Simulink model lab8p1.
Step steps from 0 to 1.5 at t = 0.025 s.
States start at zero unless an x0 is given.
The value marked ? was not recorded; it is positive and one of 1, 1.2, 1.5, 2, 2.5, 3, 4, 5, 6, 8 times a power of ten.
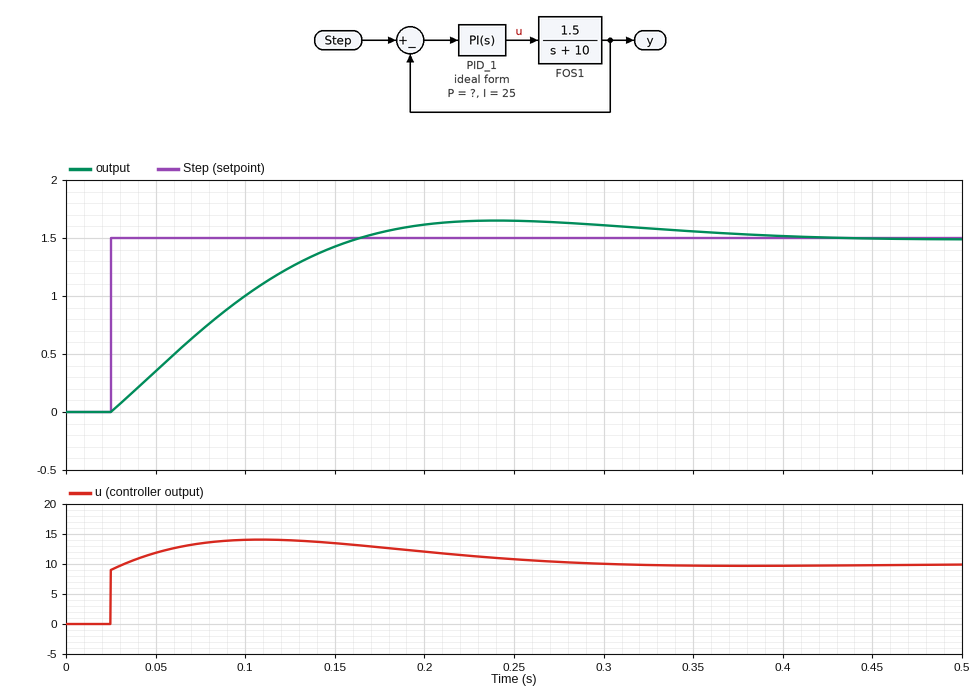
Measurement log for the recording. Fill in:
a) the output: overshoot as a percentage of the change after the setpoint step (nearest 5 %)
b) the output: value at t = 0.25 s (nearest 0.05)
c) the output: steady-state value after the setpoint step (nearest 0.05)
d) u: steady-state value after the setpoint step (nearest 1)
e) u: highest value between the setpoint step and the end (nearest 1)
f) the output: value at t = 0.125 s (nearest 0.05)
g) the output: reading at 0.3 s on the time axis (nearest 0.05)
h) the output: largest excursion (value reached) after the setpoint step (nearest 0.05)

10 %
1.65
1.50
10
14
1.25
1.60
1.65
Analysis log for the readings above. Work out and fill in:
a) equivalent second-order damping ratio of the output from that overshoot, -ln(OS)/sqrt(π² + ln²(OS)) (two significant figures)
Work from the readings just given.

0.59
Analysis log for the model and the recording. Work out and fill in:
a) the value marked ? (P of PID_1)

6
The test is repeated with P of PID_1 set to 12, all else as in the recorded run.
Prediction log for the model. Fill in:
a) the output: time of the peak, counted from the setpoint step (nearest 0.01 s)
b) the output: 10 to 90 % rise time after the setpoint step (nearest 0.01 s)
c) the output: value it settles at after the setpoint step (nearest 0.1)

0.14 s
0.06 s
1.5
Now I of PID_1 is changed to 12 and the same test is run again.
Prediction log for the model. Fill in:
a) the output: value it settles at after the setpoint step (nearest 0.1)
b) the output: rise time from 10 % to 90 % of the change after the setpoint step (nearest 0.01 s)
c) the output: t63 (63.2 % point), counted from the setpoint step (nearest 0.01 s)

1.5
0.20 s
0.10 s
